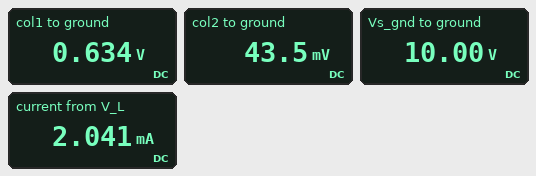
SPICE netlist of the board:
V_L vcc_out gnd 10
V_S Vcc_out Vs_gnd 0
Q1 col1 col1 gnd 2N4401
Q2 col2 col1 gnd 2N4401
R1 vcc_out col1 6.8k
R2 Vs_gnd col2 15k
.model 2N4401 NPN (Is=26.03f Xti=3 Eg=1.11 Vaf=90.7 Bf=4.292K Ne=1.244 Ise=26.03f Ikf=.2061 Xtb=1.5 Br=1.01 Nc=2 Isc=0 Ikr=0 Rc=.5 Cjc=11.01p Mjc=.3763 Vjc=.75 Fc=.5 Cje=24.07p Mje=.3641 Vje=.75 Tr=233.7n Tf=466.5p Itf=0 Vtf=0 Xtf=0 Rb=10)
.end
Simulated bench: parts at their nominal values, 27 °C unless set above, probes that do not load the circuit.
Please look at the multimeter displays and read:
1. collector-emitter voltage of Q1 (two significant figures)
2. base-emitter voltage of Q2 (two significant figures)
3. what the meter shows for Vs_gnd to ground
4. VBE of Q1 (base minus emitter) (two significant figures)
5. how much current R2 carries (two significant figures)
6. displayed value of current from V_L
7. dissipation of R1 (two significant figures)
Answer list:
630 mV
630 mV
10.00 V
630 mV
660 µA
2.041 mA
13 mW
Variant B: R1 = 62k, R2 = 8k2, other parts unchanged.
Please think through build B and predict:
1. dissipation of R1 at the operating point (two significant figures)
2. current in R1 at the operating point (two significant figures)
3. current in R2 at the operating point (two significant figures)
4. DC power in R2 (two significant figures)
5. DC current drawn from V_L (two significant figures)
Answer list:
1.4 mW
150 µA
160 µA
210 µW
310 µA
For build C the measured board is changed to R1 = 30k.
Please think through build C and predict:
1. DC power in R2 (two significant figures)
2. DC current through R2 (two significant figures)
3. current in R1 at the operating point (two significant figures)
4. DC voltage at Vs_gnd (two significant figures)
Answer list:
1.6 mW
320 µA
310 µA
10 V
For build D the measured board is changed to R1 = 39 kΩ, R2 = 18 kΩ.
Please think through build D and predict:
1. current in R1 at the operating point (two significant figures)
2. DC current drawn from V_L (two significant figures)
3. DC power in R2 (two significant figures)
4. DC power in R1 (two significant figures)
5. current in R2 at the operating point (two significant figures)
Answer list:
240 µA
490 µA
1.1 mW
2.3 mW
250 µA
